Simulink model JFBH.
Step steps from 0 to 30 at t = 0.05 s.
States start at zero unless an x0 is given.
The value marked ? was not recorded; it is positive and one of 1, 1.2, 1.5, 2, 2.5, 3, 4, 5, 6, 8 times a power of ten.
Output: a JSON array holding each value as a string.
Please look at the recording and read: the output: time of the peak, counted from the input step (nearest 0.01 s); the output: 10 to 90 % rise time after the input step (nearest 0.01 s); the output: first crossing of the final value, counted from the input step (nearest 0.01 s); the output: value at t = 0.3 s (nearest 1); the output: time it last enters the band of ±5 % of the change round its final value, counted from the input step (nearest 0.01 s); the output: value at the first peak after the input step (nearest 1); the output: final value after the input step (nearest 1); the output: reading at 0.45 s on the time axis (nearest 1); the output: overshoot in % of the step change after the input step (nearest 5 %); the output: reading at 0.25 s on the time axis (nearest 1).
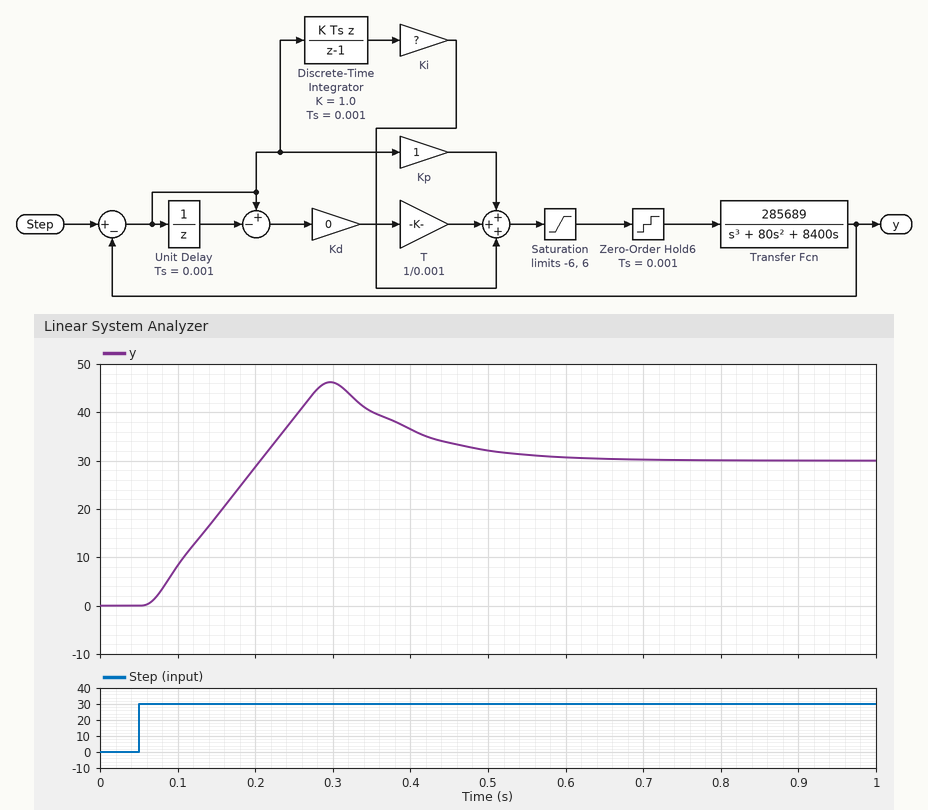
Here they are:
["0.25 s", "0.11 s", "0.16 s", "46", "0.48 s", "46", "30", "34", "55 %", "39"]
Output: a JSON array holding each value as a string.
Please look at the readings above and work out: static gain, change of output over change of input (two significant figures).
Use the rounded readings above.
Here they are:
["1.0"]
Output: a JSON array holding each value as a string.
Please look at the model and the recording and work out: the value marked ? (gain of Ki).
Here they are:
["8"]
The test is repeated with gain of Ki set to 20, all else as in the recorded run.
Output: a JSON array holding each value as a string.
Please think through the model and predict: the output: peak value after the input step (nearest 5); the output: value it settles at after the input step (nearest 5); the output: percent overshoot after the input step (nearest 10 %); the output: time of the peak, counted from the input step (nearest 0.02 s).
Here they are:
["55", "30", "80 %", "0.28 s"]
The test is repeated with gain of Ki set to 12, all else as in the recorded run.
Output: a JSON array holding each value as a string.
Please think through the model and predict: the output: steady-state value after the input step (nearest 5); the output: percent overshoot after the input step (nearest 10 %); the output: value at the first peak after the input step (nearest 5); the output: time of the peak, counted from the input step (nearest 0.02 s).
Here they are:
["30", "70 %", "50", "0.26 s"]
